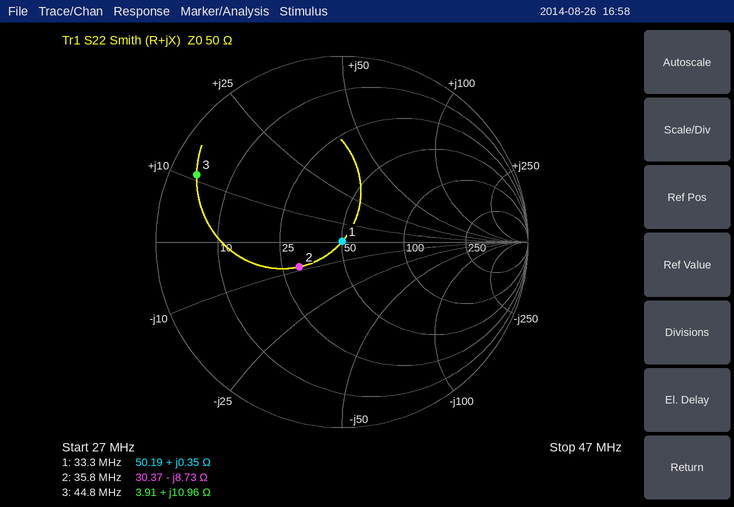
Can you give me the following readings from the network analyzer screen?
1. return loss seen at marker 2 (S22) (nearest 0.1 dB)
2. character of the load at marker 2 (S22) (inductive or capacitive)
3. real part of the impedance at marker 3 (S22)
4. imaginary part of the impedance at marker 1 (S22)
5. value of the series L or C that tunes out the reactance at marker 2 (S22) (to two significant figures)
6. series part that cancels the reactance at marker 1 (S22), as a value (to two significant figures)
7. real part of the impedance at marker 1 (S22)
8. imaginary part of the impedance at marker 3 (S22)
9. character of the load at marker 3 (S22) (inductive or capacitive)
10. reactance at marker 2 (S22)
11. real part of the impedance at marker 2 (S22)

11.5 dB
capacitive
3.91 Ω
+0.35 Ω
39 nH
14 nF
50.19 Ω
+10.96 Ω
inductive
-8.73 Ω
30.37 Ω
